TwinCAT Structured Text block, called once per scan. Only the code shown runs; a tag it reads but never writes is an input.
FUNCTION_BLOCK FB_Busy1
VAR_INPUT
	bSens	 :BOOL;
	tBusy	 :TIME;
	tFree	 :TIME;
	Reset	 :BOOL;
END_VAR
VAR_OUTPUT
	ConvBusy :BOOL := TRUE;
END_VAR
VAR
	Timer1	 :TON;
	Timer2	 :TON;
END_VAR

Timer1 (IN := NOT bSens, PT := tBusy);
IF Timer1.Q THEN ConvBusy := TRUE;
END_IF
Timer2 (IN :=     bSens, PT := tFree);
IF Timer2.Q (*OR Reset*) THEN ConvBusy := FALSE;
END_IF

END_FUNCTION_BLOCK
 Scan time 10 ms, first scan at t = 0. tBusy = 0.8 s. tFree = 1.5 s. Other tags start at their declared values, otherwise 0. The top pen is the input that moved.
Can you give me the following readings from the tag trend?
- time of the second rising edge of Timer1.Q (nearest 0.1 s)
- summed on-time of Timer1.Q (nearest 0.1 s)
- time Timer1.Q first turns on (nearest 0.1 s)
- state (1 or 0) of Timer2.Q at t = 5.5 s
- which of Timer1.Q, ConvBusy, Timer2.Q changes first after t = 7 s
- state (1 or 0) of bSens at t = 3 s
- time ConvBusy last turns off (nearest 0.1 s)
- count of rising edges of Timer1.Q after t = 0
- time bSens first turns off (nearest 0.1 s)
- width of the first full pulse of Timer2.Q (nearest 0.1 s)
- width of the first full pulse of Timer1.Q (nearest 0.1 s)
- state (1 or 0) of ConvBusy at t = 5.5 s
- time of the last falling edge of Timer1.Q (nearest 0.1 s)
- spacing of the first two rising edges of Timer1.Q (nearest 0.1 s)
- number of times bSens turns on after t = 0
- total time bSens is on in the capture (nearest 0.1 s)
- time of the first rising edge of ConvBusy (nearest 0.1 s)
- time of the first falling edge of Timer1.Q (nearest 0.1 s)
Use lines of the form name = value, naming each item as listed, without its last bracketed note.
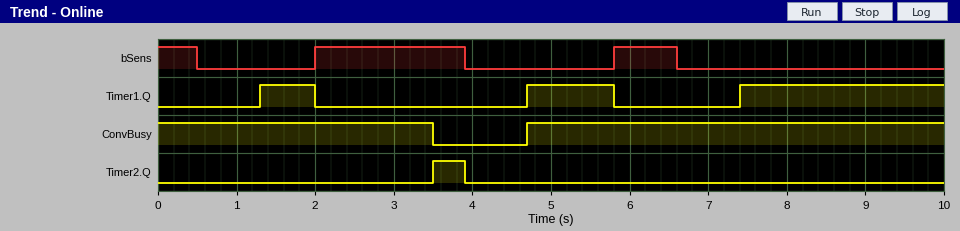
time of the second rising edge of Timer1.Q = 4.7 s
summed on-time of Timer1.Q = 4.4 s
time Timer1.Q first turns on = 1.3 s
state (1 or 0) of Timer2.Q at t = 5.5 s = 0
which of Timer1.Q, ConvBusy, Timer2.Q changes first after t = 7 s = Timer1.Q
state (1 or 0) of bSens at t = 3 s = 1
time ConvBusy last turns off = 3.5 s
count of rising edges of Timer1.Q after t = 0 = 3
time bSens first turns off = 0.5 s
width of the first full pulse of Timer2.Q = 0.4 s
width of the first full pulse of Timer1.Q = 0.7 s
state (1 or 0) of ConvBusy at t = 5.5 s = 1
time of the last falling edge of Timer1.Q = 5.8 s
spacing of the first two rising edges of Timer1.Q = 3.4 s
number of times bSens turns on after t = 0 = 2
total time bSens is on in the capture = 3.2 s
time of the first rising edge of ConvBusy = 4.7 s
time of the first falling edge of Timer1.Q = 2.0 s
